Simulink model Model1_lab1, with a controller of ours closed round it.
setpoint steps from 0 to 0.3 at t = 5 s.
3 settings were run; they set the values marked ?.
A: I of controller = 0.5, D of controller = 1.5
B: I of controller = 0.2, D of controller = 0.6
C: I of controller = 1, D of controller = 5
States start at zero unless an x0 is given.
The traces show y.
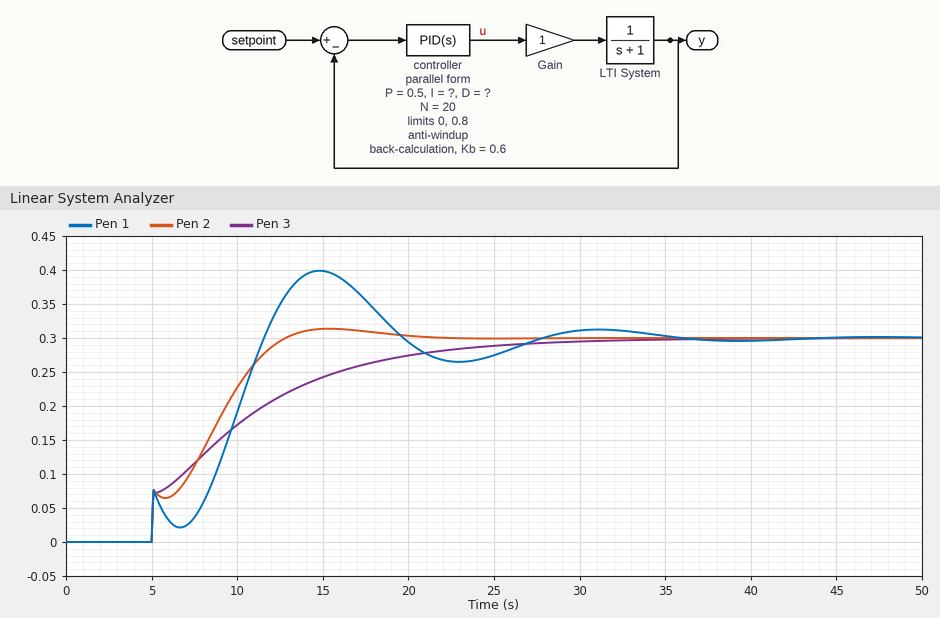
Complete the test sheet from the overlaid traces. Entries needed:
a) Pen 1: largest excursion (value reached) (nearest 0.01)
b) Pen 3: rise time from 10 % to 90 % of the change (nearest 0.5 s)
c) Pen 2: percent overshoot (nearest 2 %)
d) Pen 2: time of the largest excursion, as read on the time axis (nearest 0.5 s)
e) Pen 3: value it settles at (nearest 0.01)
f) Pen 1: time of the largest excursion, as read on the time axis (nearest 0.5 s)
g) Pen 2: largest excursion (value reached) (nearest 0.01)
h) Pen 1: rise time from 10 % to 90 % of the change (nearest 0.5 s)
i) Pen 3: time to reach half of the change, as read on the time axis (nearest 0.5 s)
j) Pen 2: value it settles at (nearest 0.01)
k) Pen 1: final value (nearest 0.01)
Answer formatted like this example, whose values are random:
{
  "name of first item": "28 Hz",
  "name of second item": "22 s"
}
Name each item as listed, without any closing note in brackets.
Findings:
{
  "Pen 1: largest excursion (value reached)": "0.40",
  "Pen 3: rise time from 10 % to 90 % of the change": "14.0 s",
  "Pen 2: percent overshoot": "4 %",
  "Pen 2: time of the largest excursion, as read on the time axis": "15.5 s",
  "Pen 3: value it settles at": "0.30",
  "Pen 1: time of the largest excursion, as read on the time axis": "15.0 s",
  "Pen 2: largest excursion (value reached)": "0.31",
  "Pen 1: rise time from 10 % to 90 % of the change": "6.0 s",
  "Pen 3: time to reach half of the change, as read on the time axis": "9.0 s",
  "Pen 2: value it settles at": "0.30",
  "Pen 1: final value": "0.30"
}
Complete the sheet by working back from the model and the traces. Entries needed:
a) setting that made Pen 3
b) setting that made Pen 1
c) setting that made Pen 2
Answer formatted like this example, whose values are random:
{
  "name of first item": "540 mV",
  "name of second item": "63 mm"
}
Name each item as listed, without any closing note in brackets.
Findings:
{
  "setting that made Pen 3": "B",
  "setting that made Pen 1": "C",
  "setting that made Pen 2": "A"
}
